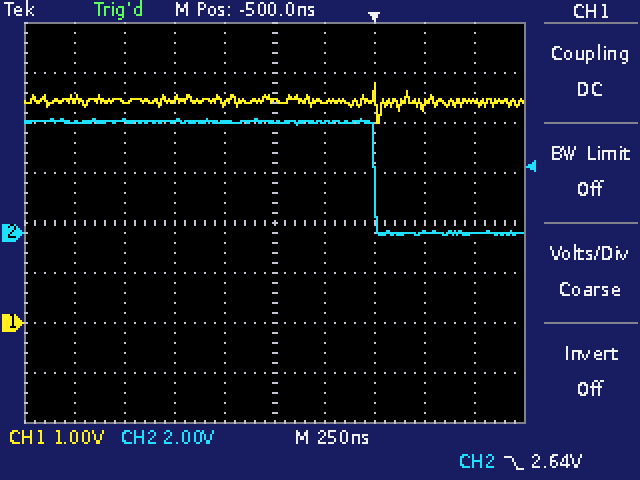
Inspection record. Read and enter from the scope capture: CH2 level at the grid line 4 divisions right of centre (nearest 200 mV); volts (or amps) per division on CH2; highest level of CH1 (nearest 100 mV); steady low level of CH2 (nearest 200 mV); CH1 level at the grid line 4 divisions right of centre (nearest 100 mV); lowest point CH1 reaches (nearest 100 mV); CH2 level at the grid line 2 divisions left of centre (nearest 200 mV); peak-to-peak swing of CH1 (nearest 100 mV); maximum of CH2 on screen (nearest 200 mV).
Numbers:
0.0 V
2 V
4.8 V
0.0 V
4.4 V
4.0 V
4.4 V
800 mV
4.6 V
